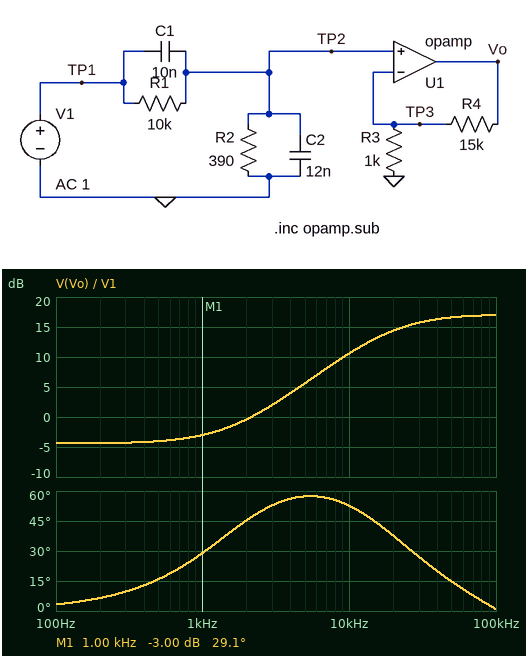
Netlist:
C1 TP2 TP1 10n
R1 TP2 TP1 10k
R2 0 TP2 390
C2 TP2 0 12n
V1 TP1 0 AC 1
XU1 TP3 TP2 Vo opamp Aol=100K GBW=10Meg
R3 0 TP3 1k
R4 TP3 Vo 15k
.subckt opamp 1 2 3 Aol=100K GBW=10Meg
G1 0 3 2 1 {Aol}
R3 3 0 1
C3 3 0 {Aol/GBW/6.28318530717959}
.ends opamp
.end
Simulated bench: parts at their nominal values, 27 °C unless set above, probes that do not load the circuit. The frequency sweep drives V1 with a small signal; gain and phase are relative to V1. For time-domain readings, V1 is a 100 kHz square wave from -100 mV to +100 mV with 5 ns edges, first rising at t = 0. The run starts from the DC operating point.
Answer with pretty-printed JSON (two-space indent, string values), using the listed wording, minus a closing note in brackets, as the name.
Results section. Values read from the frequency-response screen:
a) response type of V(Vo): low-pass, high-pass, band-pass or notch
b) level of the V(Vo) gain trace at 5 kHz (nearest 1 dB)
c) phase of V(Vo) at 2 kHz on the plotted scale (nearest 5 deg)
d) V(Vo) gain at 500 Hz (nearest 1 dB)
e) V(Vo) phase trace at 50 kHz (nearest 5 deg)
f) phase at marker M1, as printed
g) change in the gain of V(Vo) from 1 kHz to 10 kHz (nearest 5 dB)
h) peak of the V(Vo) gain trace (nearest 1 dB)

{
  "response type of V(Vo): low-pass, high-pass, band-pass or notch": "high-pass",
  "level of the V(Vo) gain trace at 5 kHz": "6 dB",
  "phase of V(Vo) at 2 kHz on the plotted scale": "45 deg",
  "V(Vo) gain at 500 Hz": "-4 dB",
  "V(Vo) phase trace at 50 kHz": "15 deg",
  "phase at marker M1, as printed": "29.1 deg",
  "change in the gain of V(Vo) from 1 kHz to 10 kHz": "15 dB",
  "peak of the V(Vo) gain trace": "17 dB"
}
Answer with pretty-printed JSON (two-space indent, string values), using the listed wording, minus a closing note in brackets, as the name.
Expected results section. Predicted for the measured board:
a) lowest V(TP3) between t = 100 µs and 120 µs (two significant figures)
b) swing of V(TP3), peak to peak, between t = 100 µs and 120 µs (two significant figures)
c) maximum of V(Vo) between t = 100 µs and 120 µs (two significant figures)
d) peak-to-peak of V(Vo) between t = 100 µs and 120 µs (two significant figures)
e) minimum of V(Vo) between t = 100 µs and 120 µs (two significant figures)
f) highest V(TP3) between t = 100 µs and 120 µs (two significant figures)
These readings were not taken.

{
  "lowest V(TP3) between t = 100 µs and 120 µs": "-51 mV",
  "swing of V(TP3), peak to peak, between t = 100 µs and 120 µs": "100 mV",
  "maximum of V(Vo) between t = 100 µs and 120 µs": "820 mV",
  "peak-to-peak of V(Vo) between t = 100 µs and 120 µs": "1.6 V",
  "minimum of V(Vo) between t = 100 µs and 120 µs": "-820 mV",
  "highest V(TP3) between t = 100 µs and 120 µs": "51 mV"
}
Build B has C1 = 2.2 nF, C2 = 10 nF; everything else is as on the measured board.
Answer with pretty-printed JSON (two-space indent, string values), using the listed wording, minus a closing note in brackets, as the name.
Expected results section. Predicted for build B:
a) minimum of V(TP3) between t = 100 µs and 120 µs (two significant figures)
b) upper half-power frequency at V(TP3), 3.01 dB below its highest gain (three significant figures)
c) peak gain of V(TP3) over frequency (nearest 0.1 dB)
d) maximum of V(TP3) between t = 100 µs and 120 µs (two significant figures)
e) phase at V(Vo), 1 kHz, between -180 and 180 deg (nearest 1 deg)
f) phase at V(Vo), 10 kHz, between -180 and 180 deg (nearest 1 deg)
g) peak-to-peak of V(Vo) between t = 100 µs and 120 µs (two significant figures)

{
  "minimum of V(TP3) between t = 100 µs and 120 µs": "-21 mV",
  "upper half-power frequency at V(TP3), 3.01 dB below its highest gain": "690 kHz",
  "peak gain of V(TP3) over frequency": "-15.3 dB",
  "maximum of V(TP3) between t = 100 µs and 120 µs": "21 mV",
  "phase at V(Vo), 1 kHz, between -180 and 180 deg": "6 deg",
  "phase at V(Vo), 10 kHz, between -180 and 180 deg": "37 deg",
  "peak-to-peak of V(Vo) between t = 100 µs and 120 µs": "680 mV"
}
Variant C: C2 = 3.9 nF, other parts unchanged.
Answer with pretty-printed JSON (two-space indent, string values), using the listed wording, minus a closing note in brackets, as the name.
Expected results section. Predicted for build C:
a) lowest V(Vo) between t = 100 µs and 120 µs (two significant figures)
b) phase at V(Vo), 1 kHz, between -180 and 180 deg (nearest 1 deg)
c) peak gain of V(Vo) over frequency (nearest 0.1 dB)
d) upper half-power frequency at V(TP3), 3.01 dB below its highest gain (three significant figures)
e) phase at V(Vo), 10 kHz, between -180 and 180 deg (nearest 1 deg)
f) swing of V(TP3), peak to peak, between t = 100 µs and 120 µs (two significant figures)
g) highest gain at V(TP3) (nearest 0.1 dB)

{
  "lowest V(Vo) between t = 100 µs and 120 µs": "-1.4 V",
  "phase at V(Vo), 1 kHz, between -180 and 180 deg": "30 deg",
  "peak gain of V(Vo) over frequency": "20.8 dB",
  "upper half-power frequency at V(TP3), 3.01 dB below its highest gain": "683 kHz",
  "phase at V(Vo), 10 kHz, between -180 and 180 deg": "62 deg",
  "swing of V(TP3), peak to peak, between t = 100 µs and 120 µs": "170 mV",
  "highest gain at V(TP3)": "-3.3 dB"
}
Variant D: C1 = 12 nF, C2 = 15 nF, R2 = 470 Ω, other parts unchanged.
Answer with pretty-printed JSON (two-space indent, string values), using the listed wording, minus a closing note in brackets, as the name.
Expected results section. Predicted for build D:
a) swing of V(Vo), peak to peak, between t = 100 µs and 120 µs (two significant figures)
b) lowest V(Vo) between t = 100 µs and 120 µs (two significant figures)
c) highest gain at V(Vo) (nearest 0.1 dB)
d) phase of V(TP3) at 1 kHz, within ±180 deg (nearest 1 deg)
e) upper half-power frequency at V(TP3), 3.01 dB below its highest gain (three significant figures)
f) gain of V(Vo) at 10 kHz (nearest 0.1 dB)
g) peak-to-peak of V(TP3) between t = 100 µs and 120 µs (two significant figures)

{
  "swing of V(Vo), peak to peak, between t = 100 µs and 120 µs": "1.5 V",
  "lowest V(Vo) between t = 100 µs and 120 µs": "-770 mV",
  "highest gain at V(Vo)": "16.9 dB",
  "phase of V(TP3) at 1 kHz, within ±180 deg": "33 deg",
  "upper half-power frequency at V(TP3), 3.01 dB below its highest gain": "651 kHz",
  "gain of V(Vo) at 10 kHz": "12.8 dB",
  "peak-to-peak of V(TP3) between t = 100 µs and 120 µs": "96 mV"
}
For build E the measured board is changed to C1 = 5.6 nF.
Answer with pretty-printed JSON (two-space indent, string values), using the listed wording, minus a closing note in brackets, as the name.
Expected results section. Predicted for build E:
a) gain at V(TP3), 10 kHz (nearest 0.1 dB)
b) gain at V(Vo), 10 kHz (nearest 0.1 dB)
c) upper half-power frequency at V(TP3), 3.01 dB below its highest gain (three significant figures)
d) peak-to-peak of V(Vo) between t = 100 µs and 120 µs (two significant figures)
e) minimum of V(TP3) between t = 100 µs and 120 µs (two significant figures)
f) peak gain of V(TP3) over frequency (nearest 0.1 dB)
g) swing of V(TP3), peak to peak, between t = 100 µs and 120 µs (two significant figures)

{
  "gain at V(TP3), 10 kHz": "-17.9 dB",
  "gain at V(Vo), 10 kHz": "6.1 dB",
  "upper half-power frequency at V(TP3), 3.01 dB below its highest gain": "671 kHz",
  "peak-to-peak of V(Vo) between t = 100 µs and 120 µs": "1.2 V",
  "minimum of V(TP3) between t = 100 µs and 120 µs": "-37 mV",
  "peak gain of V(TP3) over frequency": "-10.3 dB",
  "swing of V(TP3), peak to peak, between t = 100 µs and 120 µs": "73 mV"
}
